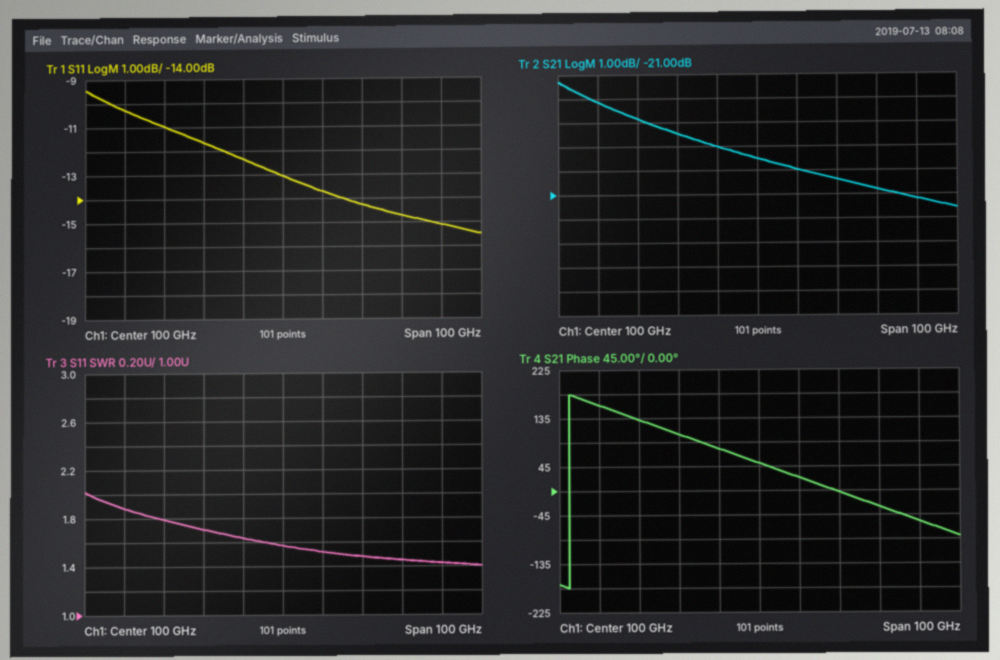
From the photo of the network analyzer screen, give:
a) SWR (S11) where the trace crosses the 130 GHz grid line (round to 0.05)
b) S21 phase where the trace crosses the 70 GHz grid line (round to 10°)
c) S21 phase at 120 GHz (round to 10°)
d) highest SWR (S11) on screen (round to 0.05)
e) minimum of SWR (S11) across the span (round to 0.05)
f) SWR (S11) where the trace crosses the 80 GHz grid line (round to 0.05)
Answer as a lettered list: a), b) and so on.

a) 1.45
b) 130°
c) 0°
d) 2.00
e) 1.40
f) 1.70
